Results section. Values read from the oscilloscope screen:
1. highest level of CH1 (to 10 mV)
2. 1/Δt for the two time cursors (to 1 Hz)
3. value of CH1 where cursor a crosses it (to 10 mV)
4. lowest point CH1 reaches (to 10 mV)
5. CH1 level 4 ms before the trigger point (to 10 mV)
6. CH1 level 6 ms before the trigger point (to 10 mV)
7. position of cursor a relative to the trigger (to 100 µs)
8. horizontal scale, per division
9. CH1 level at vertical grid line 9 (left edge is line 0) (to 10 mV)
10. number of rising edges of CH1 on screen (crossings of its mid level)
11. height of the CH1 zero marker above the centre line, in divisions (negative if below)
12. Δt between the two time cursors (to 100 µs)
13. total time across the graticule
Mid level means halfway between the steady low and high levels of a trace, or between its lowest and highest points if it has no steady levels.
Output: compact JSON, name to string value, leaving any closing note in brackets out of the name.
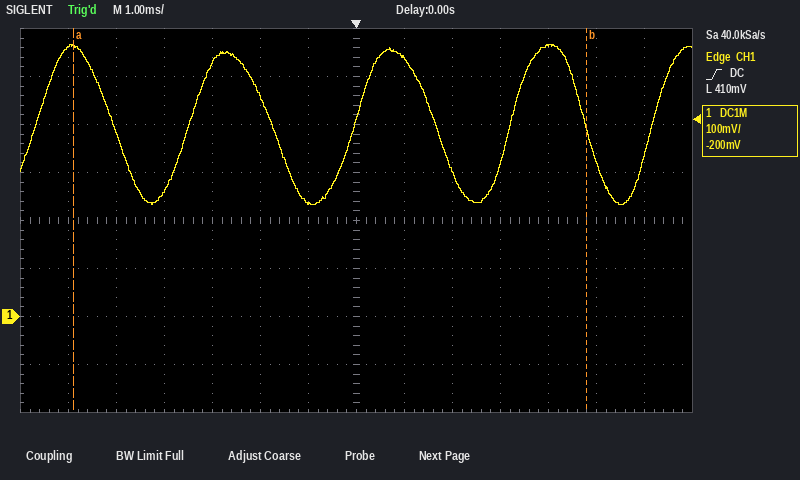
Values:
{"highest level of CH1": "570 mV", "1/Δt for the two time cursors": "93 Hz", "value of CH1 where cursor a crosses it": "560 mV", "lowest point CH1 reaches": "230 mV", "CH1 level 4 ms before the trigger point": "260 mV", "CH1 level 6 ms before the trigger point": "560 mV", "position of cursor a relative to the trigger": "-5.9 ms", "horizontal scale, per division": "1 ms", "CH1 level at vertical grid line 9 (left edge is line 0)": "300 mV", "number of rising edges of CH1 on screen": "5", "height of the CH1 zero marker above the centre line, in divisions": "-2.0 div", "Δt between the two time cursors": "10.7 ms", "total time across the graticule": "14 ms"}
